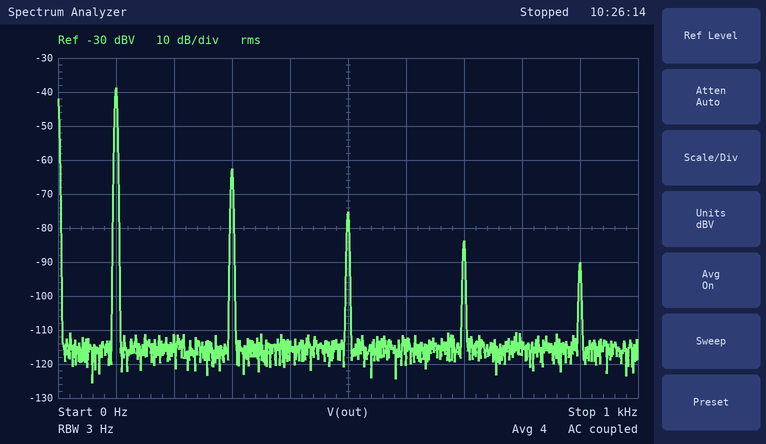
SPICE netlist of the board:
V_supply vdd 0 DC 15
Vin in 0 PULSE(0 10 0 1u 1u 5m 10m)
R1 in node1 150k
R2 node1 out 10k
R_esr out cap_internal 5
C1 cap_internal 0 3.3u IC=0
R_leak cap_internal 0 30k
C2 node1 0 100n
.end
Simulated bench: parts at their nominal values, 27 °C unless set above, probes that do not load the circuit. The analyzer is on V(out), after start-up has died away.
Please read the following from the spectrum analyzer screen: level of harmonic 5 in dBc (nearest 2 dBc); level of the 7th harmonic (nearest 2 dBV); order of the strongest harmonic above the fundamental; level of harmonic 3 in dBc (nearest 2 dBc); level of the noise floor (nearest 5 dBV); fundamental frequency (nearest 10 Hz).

-36 dBc
-84 dBV
3
-24 dBc
-115 dBV
100 Hz
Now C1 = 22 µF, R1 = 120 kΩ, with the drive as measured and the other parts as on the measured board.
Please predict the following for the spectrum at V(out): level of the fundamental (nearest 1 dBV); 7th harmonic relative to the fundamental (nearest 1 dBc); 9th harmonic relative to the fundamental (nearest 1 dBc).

-53 dBV
-44 dBc
-50 dBc
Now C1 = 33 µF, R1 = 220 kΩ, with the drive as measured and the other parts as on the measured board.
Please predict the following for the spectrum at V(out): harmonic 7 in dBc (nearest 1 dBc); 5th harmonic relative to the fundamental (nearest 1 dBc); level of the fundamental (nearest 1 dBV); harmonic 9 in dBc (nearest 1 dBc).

-43 dBc
-36 dBc
-62 dBV
-49 dBc
